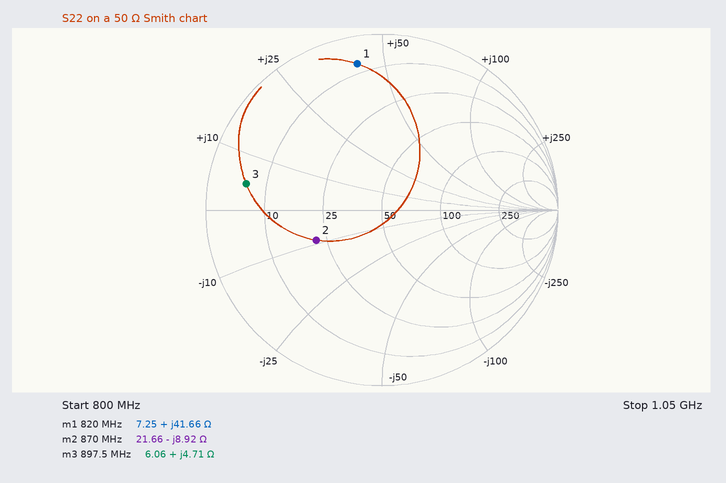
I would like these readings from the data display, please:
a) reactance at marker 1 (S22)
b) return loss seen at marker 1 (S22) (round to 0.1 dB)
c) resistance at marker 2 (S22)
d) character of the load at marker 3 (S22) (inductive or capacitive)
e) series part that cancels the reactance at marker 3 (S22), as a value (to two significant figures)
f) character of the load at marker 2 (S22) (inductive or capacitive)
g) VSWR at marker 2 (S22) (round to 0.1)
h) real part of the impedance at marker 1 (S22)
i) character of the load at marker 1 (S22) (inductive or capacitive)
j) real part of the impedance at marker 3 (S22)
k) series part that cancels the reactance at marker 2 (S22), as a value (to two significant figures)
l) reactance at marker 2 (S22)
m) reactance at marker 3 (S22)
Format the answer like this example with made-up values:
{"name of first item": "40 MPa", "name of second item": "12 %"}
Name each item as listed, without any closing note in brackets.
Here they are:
{"reactance at marker 1": "+41.66 Ω", "return loss seen at marker 1 (S22)": "1.5 dB", "resistance at marker 2": "21.66 Ω", "character of the load at marker 3 (S22)": "inductive", "series part that cancels the reactance at marker 3 (S22), as a value": "38 pF", "character of the load at marker 2 (S22)": "capacitive", "VSWR at marker 2 (S22)": "2.4", "real part of the impedance at marker 1": "7.25 Ω", "character of the load at marker 1 (S22)": "inductive", "real part of the impedance at marker 3": "6.06 Ω", "series part that cancels the reactance at marker 2 (S22), as a value": "1.6 nH", "reactance at marker 2": "-8.92 Ω", "reactance at marker 3": "+4.71 Ω"}
